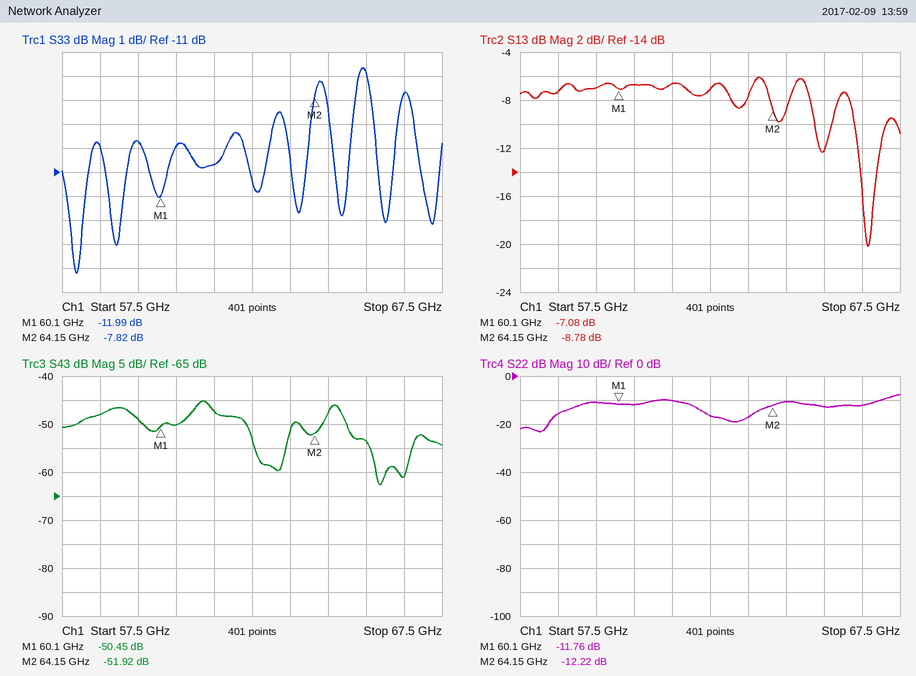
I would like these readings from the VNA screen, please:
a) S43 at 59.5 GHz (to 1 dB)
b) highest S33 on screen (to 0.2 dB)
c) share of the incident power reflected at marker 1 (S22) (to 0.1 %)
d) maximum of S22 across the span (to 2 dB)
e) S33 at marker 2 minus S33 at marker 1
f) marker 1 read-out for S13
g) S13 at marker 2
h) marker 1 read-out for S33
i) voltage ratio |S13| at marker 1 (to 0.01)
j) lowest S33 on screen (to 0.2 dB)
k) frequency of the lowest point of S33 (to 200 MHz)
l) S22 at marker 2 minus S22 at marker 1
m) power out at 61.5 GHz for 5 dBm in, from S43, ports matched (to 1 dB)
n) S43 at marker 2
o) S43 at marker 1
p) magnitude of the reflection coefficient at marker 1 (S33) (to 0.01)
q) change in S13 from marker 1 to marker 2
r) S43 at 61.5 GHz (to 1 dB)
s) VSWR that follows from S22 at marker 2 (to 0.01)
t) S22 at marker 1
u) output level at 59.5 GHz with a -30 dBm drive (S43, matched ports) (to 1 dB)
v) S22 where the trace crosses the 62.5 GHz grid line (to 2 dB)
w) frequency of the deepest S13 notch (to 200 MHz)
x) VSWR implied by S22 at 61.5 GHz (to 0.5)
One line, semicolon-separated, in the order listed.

-49 dB; -6.6 dB; 6.7 %; -8 dB; 4.17 dB; -7.08 dB; -8.78 dB; -11.99 dB; 0.44; -15.2 dB; 57.8 GHz; -0.46 dB; -42 dBm; -51.92 dB; -50.45 dB; 0.25; -1.70 dB; -47 dB; 1.65; -11.76 dB; -79 dBm; -16 dB; 66.6 GHz; 2.0
